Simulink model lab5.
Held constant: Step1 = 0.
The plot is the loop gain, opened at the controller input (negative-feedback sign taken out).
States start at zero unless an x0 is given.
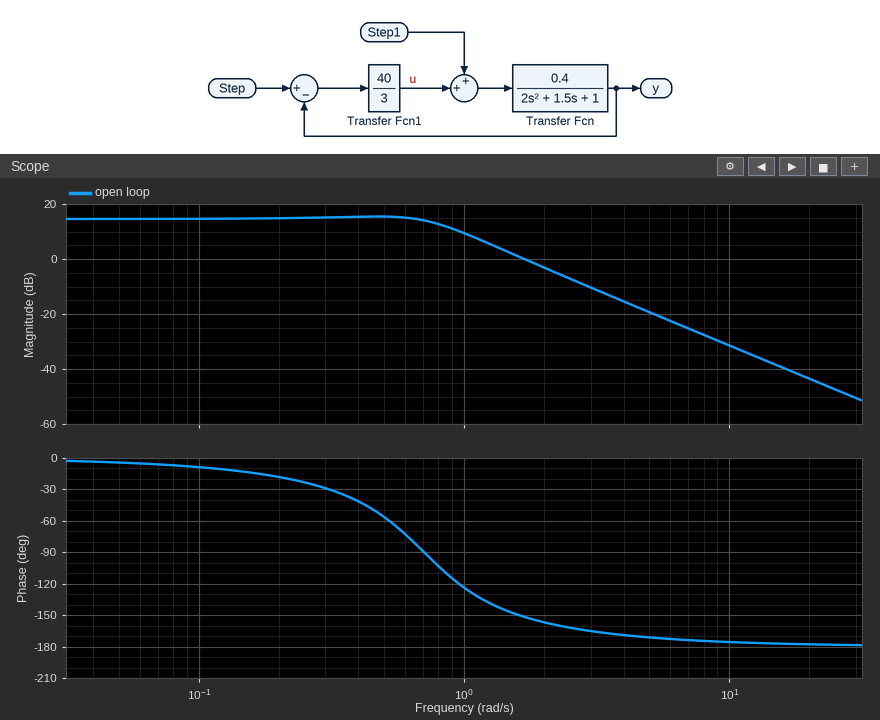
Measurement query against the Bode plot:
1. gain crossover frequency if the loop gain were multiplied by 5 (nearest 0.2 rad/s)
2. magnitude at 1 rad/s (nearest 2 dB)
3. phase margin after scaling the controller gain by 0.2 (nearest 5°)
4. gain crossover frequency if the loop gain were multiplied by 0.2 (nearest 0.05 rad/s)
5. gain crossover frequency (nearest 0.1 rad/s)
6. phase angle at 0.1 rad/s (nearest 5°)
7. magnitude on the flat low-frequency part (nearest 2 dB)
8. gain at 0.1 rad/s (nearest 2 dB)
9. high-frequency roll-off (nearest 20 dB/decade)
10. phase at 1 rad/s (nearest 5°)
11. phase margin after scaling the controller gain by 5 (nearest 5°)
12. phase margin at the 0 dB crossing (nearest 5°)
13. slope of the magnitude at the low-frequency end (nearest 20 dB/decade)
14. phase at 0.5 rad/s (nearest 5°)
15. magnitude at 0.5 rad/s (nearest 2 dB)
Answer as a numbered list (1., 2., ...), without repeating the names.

1. 3.6 rad/s
2. 10 dB
3. 90°
4. 0.70 rad/s
5. 1.7 rad/s
6. -10°
7. 14 dB
8. 14 dB
9. -40 dB/decade
10. -125°
11. 10°
12. 30°
13. 0 dB/decade
14. -55°
15. 16 dB
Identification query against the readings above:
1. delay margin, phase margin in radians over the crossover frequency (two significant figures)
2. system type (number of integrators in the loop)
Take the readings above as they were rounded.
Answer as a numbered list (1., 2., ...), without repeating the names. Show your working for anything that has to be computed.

1. 30 × π / 180 / 1.7 = 0.31 s
2. 0
